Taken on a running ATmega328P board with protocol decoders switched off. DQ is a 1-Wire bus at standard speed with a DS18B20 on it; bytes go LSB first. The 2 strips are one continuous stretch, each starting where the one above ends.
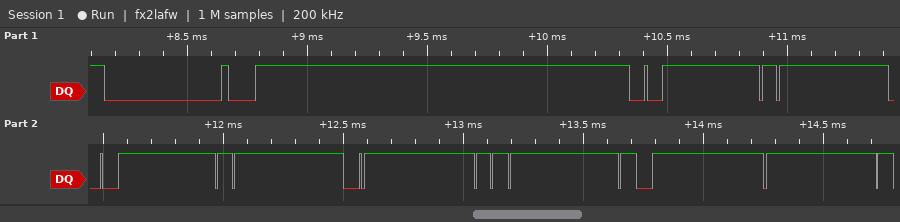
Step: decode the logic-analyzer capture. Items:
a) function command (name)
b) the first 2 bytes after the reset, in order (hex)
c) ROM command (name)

Read Scratchpad
CC BE
Skip ROM
